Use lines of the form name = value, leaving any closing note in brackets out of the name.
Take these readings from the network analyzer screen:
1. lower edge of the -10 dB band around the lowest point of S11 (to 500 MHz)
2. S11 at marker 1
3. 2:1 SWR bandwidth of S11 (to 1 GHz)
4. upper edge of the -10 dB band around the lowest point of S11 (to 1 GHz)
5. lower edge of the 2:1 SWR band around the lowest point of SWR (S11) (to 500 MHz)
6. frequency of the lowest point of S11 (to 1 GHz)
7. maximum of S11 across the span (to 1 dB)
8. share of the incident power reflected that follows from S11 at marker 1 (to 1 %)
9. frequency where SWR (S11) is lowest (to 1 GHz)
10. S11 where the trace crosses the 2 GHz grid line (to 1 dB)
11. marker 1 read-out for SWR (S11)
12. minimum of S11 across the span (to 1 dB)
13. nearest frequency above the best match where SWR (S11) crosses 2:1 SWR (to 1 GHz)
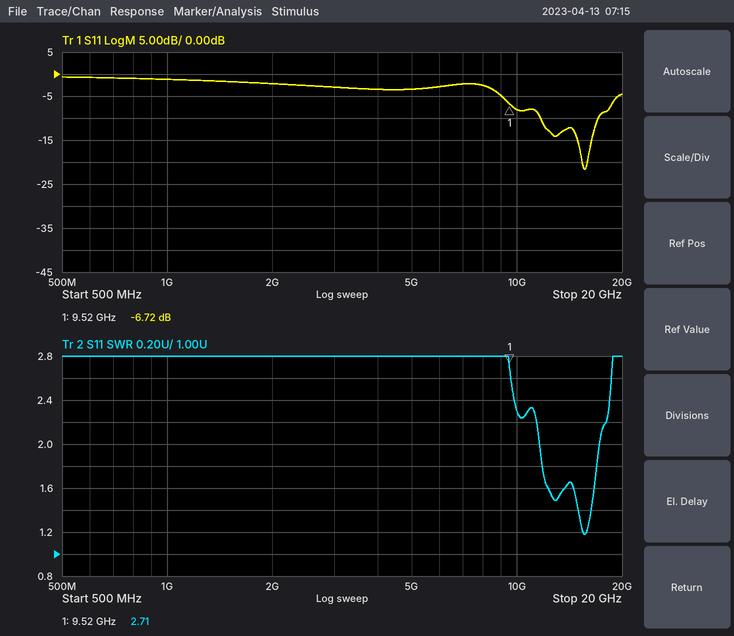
lower edge of the -10 dB band around the lowest point of S11 = 11.5 GHz
S11 at marker 1 = -6.72 dB
2:1 SWR bandwidth of S11 = 6 GHz
upper edge of the -10 dB band around the lowest point of S11 = 17 GHz
lower edge of the 2:1 SWR band around the lowest point of SWR (S11) = 11.5 GHz
frequency of the lowest point of S11 = 16 GHz
maximum of S11 across the span = -1 dB
share of the incident power reflected that follows from S11 at marker 1 = 21 %
frequency where SWR (S11) is lowest = 16 GHz
S11 where the trace crosses the 2 GHz grid line = -2 dB
marker 1 read-out for SWR = 2.71
minimum of S11 across the span = -22 dB
nearest frequency above the best match where SWR (S11) crosses 2:1 SWR = 17 GHz
